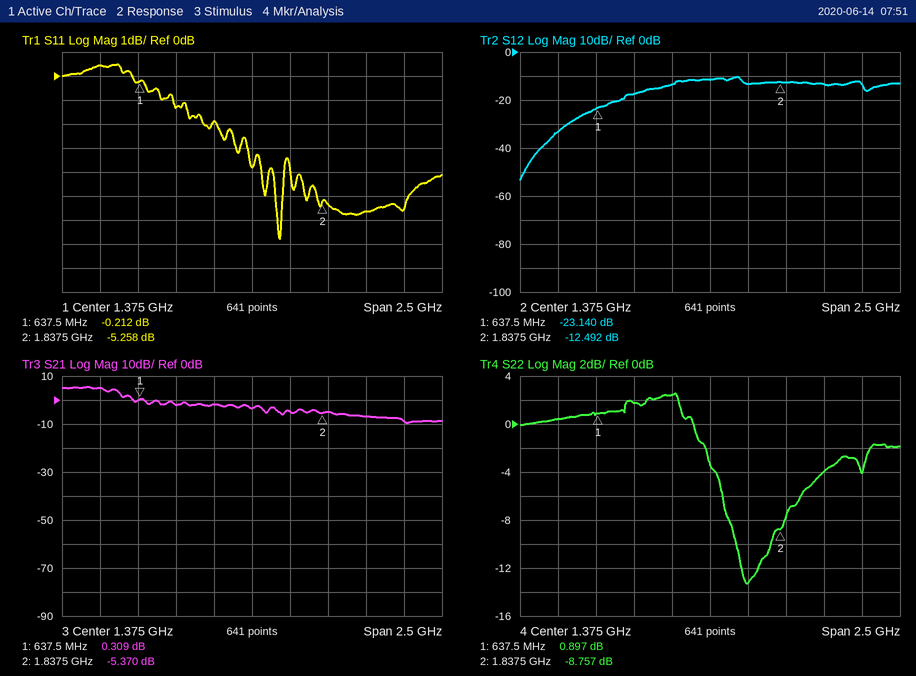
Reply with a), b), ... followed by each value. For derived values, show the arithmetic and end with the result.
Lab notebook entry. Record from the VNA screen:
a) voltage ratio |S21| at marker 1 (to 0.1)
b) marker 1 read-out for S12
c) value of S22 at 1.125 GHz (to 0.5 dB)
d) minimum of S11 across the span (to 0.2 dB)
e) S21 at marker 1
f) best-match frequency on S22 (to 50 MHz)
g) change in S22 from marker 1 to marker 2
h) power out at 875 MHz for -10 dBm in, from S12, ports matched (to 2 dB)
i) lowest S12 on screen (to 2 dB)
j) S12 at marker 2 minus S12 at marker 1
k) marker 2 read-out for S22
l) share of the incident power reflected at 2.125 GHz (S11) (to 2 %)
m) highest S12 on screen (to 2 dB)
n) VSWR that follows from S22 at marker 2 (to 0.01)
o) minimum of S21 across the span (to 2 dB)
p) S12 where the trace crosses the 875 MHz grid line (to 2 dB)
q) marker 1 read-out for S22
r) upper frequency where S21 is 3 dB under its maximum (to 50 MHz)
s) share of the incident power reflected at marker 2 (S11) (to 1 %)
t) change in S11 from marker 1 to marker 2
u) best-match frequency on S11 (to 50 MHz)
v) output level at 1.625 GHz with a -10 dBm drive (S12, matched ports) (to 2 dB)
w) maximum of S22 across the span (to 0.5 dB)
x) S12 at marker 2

a) 10^(0.309/20) ≈ 1.0
b) -23.140 dB
c) 2.5 dB
d) -6.8 dB
e) 0.309 dB
f) 1.60 GHz
g) -8.757 − (0.897) = -9.654 dB
h) -10 dBm + (-18 dB) = -28 dBm
i) -54 dB
j) -12.492 − (-23.14) = 10.648 dB
k) -8.757 dB
l) 10^(-5.6/10) ≈ 28 %
m) -10 dB
n) (1 + 0.3649)/(1 − 0.3649) ≈ 2.15
o) -10 dB
p) -18 dB
q) 0.897 dB
r) 500 MHz
s) 10^(-5.258/10) ≈ 30 %
t) -5.258 − (-0.212) = -5.046 dB
u) 1.55 GHz
v) -10 dBm + (-14 dB) = -24 dBm
w) 2.5 dB
x) -12.492 dB
